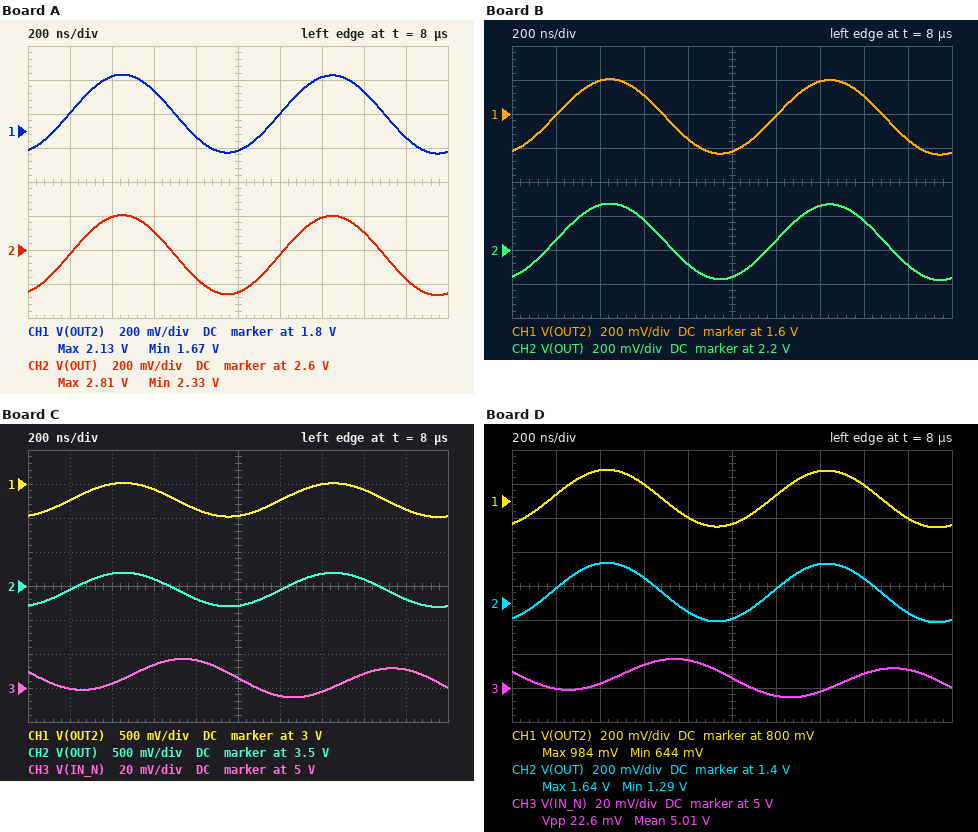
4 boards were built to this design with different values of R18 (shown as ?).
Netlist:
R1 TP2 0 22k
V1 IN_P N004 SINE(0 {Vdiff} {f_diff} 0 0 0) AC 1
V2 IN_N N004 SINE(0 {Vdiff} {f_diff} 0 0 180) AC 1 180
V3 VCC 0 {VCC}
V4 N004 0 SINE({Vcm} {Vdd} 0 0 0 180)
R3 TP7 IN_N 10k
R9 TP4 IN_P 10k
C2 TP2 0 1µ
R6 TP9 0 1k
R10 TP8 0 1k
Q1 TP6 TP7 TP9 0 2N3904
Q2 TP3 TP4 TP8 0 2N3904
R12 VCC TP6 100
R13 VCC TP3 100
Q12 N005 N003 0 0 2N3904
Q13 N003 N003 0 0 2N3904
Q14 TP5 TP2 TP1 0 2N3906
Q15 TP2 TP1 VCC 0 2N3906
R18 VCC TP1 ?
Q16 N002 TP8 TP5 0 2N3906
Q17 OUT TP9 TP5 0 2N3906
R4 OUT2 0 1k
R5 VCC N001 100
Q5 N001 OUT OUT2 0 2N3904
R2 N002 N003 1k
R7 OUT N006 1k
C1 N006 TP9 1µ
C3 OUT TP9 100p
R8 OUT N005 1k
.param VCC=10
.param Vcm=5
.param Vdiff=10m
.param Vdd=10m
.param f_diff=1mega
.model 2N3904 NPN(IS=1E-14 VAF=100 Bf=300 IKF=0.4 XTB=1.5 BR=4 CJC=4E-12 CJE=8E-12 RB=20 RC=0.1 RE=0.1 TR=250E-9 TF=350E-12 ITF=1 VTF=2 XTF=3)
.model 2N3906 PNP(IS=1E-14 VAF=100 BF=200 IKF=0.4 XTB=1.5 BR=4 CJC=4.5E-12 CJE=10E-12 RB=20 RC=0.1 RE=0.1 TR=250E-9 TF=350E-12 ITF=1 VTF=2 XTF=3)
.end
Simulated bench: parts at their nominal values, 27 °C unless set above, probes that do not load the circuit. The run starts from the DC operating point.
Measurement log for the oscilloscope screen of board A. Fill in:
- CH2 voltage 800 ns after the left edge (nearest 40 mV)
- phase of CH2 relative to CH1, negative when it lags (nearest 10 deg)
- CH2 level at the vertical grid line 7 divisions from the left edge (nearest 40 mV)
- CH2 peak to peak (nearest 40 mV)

2.44 V
0 deg
2.80 V
480 mV
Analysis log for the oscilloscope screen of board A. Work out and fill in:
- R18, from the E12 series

180 Ω
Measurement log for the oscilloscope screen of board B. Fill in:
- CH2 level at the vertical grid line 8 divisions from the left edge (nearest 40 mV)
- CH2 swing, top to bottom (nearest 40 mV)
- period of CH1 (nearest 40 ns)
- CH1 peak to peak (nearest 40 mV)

2.36 V
440 mV
1.00 µs
440 mV
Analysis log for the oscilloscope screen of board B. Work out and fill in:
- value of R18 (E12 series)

220 Ω
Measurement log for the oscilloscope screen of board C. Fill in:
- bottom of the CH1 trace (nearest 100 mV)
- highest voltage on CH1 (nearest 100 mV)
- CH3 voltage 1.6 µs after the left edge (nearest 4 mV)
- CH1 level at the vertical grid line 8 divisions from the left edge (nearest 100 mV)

2.5 V
3.0 V
5.008 V
2.9 V
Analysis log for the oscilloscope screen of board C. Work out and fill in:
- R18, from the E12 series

120 Ω
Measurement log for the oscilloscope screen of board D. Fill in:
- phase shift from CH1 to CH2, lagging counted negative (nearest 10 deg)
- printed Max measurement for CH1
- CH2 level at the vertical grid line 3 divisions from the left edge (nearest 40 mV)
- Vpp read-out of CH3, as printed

0 deg
984 mV
1.56 V
22.6 mV
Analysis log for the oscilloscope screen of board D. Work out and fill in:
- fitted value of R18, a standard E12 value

470 Ω
